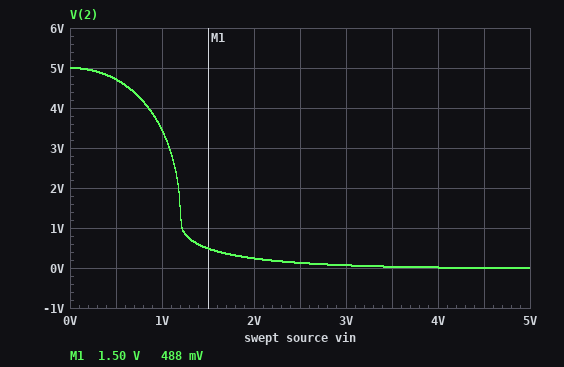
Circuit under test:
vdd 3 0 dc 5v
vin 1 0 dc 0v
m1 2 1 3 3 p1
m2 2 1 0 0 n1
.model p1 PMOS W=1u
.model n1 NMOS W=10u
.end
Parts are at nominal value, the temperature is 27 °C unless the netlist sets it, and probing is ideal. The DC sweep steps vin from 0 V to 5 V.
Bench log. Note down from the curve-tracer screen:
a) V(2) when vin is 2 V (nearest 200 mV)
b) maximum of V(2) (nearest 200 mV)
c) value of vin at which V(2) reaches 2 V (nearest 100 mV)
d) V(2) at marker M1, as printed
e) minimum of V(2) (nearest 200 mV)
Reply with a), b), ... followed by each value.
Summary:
a) 200 mV
b) 5.0 V
c) 1.2 V
d) 488 mV
e) 0 V
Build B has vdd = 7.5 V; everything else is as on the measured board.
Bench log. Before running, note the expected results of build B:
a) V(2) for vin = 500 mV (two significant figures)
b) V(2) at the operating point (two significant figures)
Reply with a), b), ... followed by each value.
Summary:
a) 7.3 V
b) 7.5 V
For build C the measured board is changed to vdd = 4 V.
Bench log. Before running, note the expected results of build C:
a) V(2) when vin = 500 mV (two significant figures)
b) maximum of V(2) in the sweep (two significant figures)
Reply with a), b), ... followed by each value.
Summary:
a) 3.6 V
b) 4.0 V
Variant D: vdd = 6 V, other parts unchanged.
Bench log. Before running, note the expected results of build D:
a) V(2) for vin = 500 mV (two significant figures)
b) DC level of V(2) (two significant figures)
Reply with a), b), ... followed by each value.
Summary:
a) 5.8 V
b) 6.0 V
